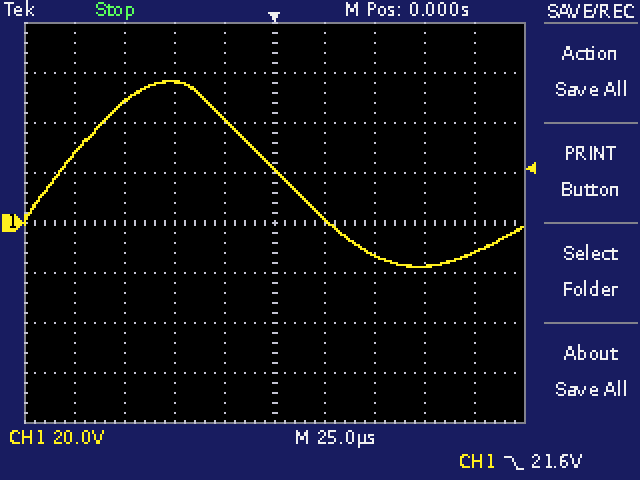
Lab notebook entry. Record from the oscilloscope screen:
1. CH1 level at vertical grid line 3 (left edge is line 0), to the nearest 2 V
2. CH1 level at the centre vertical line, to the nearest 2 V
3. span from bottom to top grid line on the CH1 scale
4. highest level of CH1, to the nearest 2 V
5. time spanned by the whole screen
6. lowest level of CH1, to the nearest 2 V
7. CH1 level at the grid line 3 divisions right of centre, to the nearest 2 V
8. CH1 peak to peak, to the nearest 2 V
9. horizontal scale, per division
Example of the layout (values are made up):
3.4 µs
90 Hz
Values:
56 V
22 V
160 V
56 V
250 µs
-18 V
-18 V
74 V
25 µs
